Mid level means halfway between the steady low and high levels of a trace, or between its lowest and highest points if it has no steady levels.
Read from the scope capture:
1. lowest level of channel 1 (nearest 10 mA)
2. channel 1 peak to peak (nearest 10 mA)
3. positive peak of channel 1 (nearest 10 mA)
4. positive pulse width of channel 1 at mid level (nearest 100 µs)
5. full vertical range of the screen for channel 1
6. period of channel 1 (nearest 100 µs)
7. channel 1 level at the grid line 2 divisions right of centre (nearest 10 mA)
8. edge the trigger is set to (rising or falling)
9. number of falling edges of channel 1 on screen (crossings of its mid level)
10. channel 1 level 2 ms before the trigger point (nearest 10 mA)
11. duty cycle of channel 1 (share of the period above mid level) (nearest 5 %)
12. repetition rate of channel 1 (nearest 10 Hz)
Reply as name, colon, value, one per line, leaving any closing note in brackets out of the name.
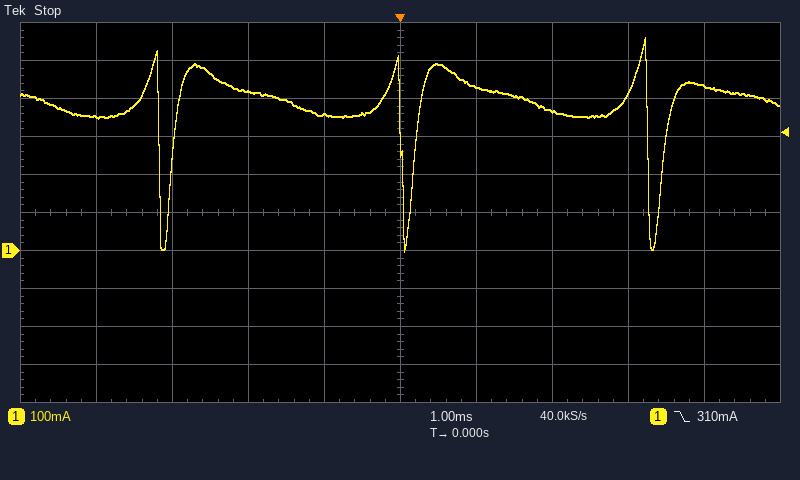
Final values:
lowest level of channel 1: 0 mA
channel 1 peak to peak: 560 mA
positive peak of channel 1: 560 mA
positive pulse width of channel 1 at mid level: 3.0 ms
full vertical range of the screen for channel 1: 1 A
period of channel 1: 3.2 ms
channel 1 level at the grid line 2 divisions right of centre: 370 mA
edge the trigger is set to: falling
number of falling edges of channel 1 on screen: 3
channel 1 level 2 ms before the trigger point: 420 mA
duty cycle of channel 1 (share of the period above mid level): 95 %
repetition rate of channel 1: 310 Hz
